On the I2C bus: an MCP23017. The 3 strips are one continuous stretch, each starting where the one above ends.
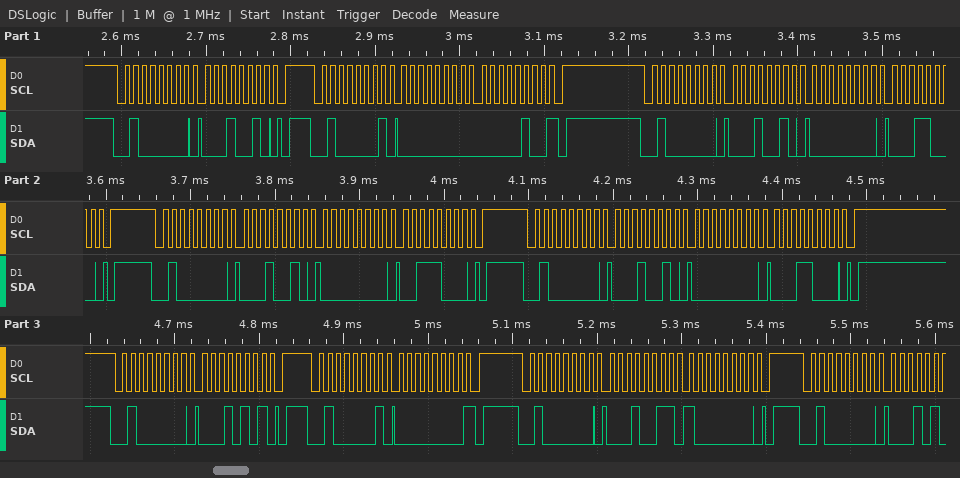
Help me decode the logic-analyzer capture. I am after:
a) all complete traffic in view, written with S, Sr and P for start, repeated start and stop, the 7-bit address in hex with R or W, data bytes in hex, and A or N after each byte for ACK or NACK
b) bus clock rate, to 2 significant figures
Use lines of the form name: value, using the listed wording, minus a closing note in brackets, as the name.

all complete traffic in view, written with S, Sr and P for start, repeated start and stop, the 7-bit address in hex with R or W, data bytes in hex, and A or N after each byte for ACK or NACK: S 20W A 12 A P S 20R A 00 A 04 N P S 20W A 12 A 00 A 18 A P S 20W A 12 A 00 A 38 A P S 20W A 12 A 00 A 18 A P S 20W A 15 A P S 20R A 00 N P S 20W A 13 A 80 A P S 20W A
bus clock rate, to 2 significant figures: 100 kHz
